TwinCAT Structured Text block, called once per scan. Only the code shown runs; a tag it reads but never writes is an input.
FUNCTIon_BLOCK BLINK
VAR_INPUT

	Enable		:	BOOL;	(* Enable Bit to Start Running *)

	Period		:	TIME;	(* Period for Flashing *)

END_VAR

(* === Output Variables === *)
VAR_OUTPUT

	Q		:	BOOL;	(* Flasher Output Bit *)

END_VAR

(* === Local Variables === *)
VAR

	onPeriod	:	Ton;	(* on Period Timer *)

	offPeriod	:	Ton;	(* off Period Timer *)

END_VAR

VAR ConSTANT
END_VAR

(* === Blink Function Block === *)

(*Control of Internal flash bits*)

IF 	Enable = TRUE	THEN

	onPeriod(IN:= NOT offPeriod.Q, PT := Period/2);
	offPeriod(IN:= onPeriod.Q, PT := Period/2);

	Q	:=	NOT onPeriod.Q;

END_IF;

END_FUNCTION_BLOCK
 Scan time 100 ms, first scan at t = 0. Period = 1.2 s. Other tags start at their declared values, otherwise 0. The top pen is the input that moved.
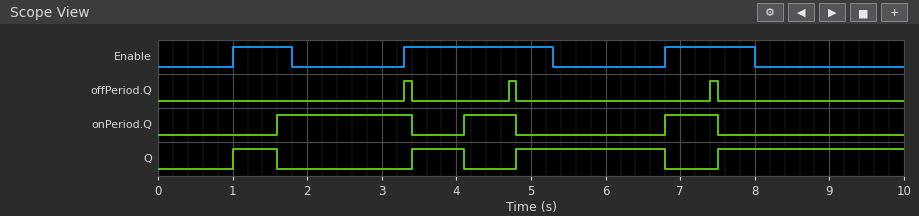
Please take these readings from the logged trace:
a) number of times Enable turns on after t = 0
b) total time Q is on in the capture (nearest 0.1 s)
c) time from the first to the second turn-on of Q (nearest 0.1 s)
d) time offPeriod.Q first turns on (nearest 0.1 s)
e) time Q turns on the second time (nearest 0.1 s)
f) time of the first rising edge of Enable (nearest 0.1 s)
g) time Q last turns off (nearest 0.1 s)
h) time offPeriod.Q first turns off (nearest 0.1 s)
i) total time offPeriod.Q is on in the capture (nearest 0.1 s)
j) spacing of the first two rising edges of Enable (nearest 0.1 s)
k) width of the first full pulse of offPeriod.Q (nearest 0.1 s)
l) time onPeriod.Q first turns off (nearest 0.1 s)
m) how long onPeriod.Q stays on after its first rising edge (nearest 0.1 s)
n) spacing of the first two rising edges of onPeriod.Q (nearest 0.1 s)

3
5.8 s
2.4 s
3.3 s
3.4 s
1.0 s
6.8 s
3.4 s
0.3 s
2.3 s
0.1 s
3.4 s
1.8 s
2.5 s
